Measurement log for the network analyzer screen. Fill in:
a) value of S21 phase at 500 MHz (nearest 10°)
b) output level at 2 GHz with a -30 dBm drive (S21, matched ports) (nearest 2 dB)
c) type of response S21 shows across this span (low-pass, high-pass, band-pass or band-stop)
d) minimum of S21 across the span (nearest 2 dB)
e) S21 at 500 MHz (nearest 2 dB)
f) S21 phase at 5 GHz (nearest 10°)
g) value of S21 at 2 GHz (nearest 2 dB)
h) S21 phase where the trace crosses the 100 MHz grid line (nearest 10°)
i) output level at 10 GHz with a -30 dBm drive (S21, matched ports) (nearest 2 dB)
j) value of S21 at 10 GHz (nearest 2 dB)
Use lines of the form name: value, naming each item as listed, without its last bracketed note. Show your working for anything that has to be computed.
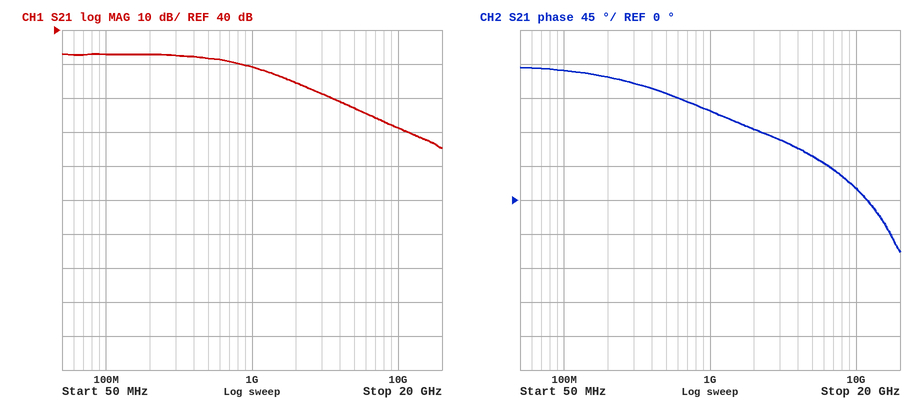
value of S21 phase at 500 MHz: 140°
output level at 2 GHz with a -30 dBm drive (S21, matched ports): -30 dBm + (24 dB) = -6 dBm
type of response S21 shows across this span: low-pass
minimum of S21 across the span: 6 dB
S21 at 500 MHz: 32 dB
S21 phase at 5 GHz: 60°
value of S21 at 2 GHz: 24 dB
S21 phase where the trace crosses the 100 MHz grid line: 170°
output level at 10 GHz with a -30 dBm drive (S21, matched ports): -30 dBm + (12 dB) = -18 dBm
value of S21 at 10 GHz: 12 dB
